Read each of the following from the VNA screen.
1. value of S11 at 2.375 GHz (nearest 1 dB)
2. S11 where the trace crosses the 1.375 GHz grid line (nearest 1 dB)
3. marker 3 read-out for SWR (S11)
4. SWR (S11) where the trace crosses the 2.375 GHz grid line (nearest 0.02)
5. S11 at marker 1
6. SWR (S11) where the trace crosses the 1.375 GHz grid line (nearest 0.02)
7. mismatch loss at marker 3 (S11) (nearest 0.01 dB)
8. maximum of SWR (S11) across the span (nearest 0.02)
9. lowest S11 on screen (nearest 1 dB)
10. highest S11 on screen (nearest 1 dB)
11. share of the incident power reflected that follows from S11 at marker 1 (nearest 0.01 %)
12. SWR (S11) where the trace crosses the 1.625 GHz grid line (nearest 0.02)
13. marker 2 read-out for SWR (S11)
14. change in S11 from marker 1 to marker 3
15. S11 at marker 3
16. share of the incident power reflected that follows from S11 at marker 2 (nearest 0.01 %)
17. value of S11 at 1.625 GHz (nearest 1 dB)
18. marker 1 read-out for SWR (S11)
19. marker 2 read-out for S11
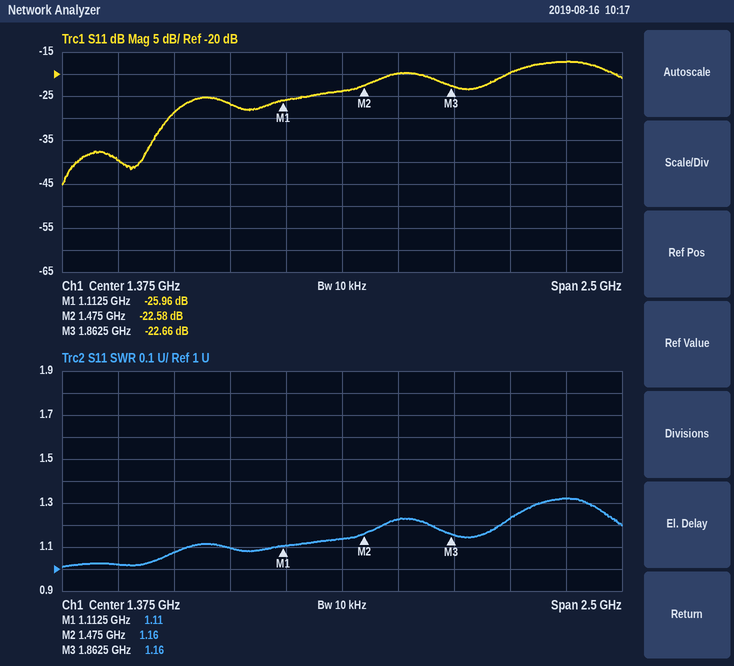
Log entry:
-17 dB
-24 dB
1.16
1.32
-25.96 dB
1.14
0.02 dB
1.32
-45 dB
-17 dB
0.25 %
1.22
1.16
3.30 dB
-22.66 dB
0.55 %
-20 dB
1.11
-22.58 dB
